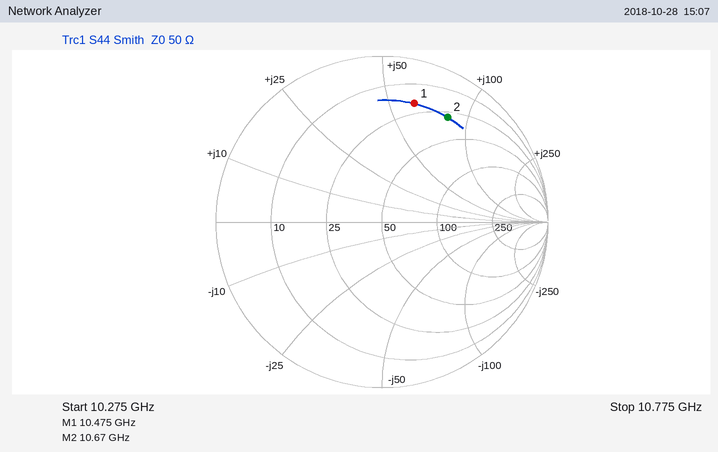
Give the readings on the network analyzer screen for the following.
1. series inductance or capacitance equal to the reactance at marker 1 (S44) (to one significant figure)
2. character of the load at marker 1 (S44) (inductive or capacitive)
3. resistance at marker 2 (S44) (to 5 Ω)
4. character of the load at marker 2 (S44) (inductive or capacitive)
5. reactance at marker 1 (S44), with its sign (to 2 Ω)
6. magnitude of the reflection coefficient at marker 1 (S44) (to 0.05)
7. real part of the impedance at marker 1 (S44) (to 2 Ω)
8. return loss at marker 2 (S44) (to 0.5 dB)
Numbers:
900 pH
inductive
30 Ω
inductive
+62 Ω
0.75
20 Ω
2.5 dB
